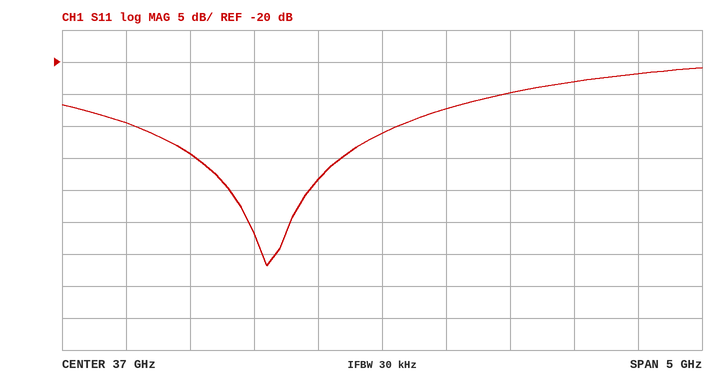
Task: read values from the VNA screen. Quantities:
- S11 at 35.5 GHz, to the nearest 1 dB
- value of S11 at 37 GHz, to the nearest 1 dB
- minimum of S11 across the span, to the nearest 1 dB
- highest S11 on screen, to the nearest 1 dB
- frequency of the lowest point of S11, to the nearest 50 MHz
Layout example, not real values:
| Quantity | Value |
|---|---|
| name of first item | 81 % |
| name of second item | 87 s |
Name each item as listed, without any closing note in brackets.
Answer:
| Quantity | Value |
|---|---|
| S11 at 35.5 GHz, to the nearest 1 dB | -34 dB |
| value of S11 at 37 GHz, to the nearest 1 dB | -31 dB |
| minimum of S11 across the span, to the nearest 1 dB | -52 dB |
| highest S11 on screen, to the nearest 1 dB | -21 dB |
| frequency of the lowest point of S11, to the nearest 50 MHz | 36.10 GHz |
